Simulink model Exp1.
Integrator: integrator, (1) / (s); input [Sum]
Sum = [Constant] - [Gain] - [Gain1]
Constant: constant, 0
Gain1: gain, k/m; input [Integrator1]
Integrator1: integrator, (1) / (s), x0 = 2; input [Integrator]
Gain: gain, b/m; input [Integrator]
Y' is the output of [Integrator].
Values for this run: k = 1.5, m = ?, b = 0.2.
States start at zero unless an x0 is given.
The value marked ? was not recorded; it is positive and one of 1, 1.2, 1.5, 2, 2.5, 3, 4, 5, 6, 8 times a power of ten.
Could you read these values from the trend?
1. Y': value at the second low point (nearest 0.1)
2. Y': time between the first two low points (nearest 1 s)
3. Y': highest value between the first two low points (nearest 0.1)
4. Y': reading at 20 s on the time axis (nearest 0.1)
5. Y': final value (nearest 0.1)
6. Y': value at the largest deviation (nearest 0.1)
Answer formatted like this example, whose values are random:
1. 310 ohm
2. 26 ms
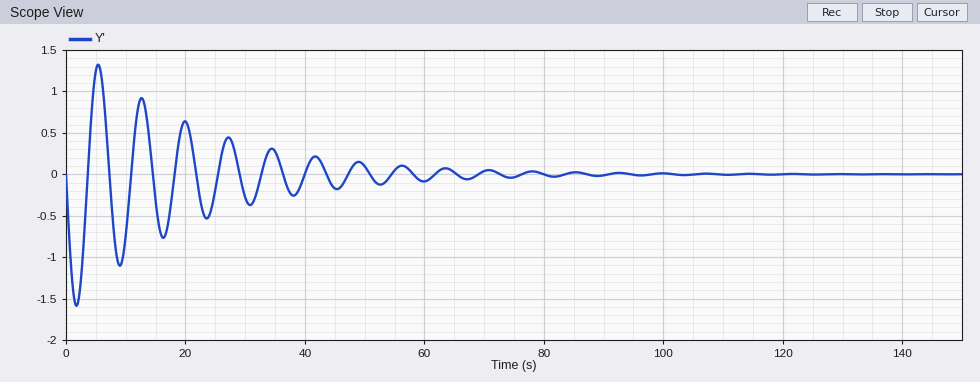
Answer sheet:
1. -1.1
2. 7 s
3. 1.3
4. 0.6
5. 0.0
6. -1.6
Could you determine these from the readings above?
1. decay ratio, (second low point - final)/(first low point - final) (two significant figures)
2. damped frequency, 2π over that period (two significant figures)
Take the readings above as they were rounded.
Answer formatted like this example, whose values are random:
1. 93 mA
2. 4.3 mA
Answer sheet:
1. 0.69
2. 0.90 rad/s
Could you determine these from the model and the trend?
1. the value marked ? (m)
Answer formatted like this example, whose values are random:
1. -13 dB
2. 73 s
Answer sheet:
1. 2
